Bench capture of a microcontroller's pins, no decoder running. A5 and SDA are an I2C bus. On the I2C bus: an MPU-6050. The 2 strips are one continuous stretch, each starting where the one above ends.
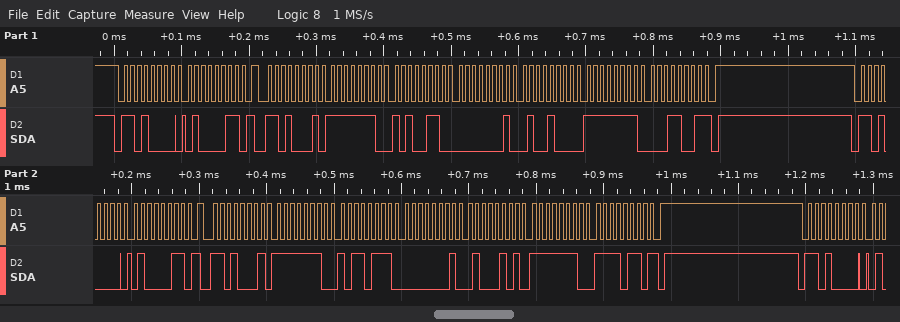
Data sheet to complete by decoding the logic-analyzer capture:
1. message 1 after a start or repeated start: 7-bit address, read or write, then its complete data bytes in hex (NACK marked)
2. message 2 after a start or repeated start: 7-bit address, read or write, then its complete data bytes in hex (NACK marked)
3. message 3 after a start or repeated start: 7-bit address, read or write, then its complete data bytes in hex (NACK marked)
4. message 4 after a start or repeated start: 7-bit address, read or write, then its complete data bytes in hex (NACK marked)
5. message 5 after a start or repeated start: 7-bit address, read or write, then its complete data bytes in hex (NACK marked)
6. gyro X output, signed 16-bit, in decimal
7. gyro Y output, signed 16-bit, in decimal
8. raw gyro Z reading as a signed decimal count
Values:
0x68 write: 43
0x68 read: FE A6 01 48 FF 19 NACK
0x68 write: 43
0x68 read: FE B7 01 45 FE F6 NACK
0x68 write
-346
328
-231
